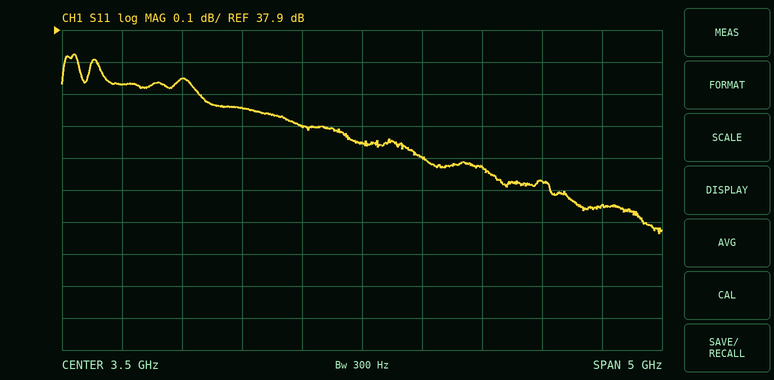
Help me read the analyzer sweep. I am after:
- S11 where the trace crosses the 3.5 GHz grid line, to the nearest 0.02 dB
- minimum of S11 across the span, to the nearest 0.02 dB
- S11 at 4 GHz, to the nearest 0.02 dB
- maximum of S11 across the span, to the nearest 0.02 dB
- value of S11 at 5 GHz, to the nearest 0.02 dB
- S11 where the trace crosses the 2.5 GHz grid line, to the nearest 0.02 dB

37.54 dB
37.26 dB
37.50 dB
37.82 dB
37.42 dB
37.66 dB
